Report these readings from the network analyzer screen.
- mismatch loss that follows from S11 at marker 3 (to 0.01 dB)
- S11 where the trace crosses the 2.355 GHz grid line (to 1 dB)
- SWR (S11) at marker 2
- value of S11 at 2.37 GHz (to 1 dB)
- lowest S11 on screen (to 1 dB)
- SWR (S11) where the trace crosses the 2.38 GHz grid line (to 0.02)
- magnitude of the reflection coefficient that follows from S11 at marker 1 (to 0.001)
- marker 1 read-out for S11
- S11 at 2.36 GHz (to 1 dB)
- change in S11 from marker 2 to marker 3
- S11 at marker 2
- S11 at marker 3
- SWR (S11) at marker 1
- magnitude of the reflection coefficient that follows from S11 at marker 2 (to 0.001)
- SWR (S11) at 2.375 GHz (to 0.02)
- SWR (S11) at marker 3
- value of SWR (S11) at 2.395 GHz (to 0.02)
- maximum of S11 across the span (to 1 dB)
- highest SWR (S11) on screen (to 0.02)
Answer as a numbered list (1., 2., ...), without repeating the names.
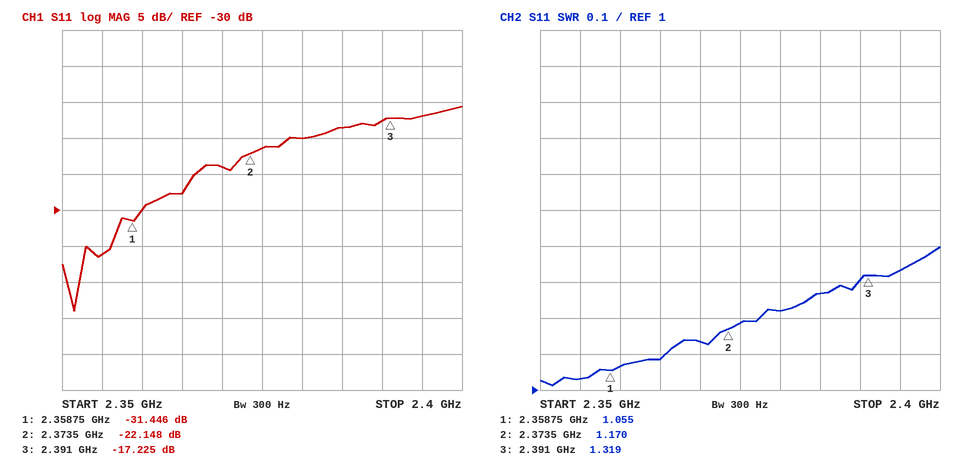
1. 0.08 dB
2. -36 dB
3. 1.170
4. -24 dB
5. -44 dB
6. 1.22
7. 0.027
8. -31.446 dB
9. -30 dB
10. 4.923 dB
11. -22.148 dB
12. -17.225 dB
13. 1.055
14. 0.078
15. 1.18
16. 1.319
17. 1.34
18. -16 dB
19. 1.40
